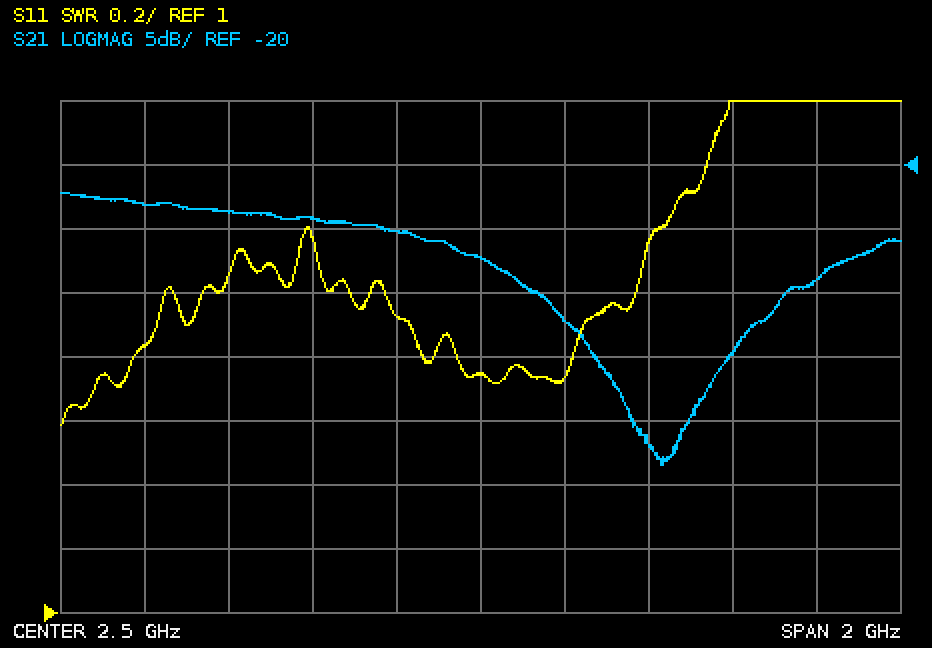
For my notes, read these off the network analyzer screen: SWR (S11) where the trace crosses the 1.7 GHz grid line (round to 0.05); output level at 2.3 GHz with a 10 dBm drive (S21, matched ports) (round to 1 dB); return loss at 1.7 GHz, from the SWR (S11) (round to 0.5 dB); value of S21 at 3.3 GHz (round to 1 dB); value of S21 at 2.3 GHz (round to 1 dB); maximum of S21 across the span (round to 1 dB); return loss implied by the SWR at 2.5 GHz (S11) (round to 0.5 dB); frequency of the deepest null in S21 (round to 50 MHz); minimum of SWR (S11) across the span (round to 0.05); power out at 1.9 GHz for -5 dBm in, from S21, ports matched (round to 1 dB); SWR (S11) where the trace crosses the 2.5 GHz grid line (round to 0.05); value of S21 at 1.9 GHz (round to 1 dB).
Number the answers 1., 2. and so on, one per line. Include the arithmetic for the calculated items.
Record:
1. 1.85
2. 10 dBm + (-25 dB) = -15 dBm
3. −20 log10((1.85 − 1)/(1.85 + 1)) ≈ 10.5 dB
4. -29 dB
5. -25 dB
6. -22 dB
7. −20 log10((1.75 − 1)/(1.75 + 1)) ≈ 11.3 dB, so 11.5 dB to the nearest 0.5 dB
8. 2.95 GHz
9. 1.60
10. -5 dBm + (-24 dB) = -29 dBm
11. 1.75
12. -24 dB
